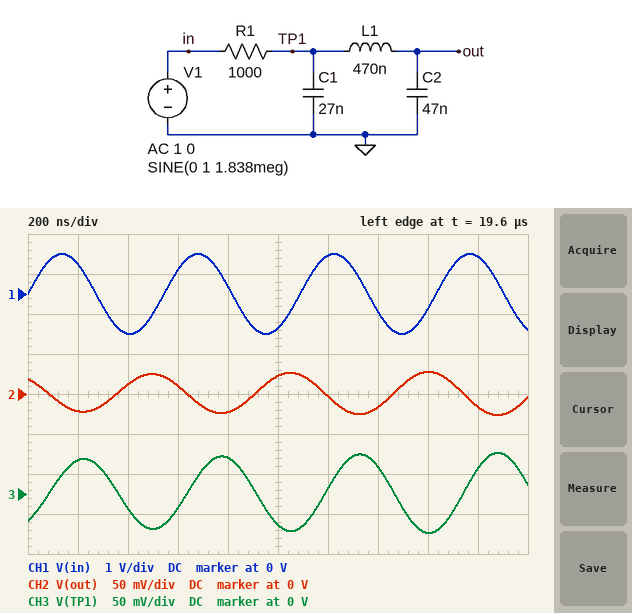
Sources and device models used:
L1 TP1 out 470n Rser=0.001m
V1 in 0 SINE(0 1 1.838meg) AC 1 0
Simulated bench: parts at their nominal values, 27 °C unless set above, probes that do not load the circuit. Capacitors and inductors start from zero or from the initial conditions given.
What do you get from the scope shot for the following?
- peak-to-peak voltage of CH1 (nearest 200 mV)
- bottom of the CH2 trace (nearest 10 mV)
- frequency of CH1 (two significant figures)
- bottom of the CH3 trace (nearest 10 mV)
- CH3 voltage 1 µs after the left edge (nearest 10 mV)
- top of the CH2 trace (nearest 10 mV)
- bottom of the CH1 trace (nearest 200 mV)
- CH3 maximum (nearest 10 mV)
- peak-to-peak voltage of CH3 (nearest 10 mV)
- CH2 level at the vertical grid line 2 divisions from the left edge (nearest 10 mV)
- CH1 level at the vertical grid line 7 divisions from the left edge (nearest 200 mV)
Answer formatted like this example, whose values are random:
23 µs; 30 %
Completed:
2.0 V; -30 mV; 1.8 MHz; -50 mV; -40 mV; 30 mV; -1.0 V; 50 mV; 100 mV; 10 mV; -400 mV
